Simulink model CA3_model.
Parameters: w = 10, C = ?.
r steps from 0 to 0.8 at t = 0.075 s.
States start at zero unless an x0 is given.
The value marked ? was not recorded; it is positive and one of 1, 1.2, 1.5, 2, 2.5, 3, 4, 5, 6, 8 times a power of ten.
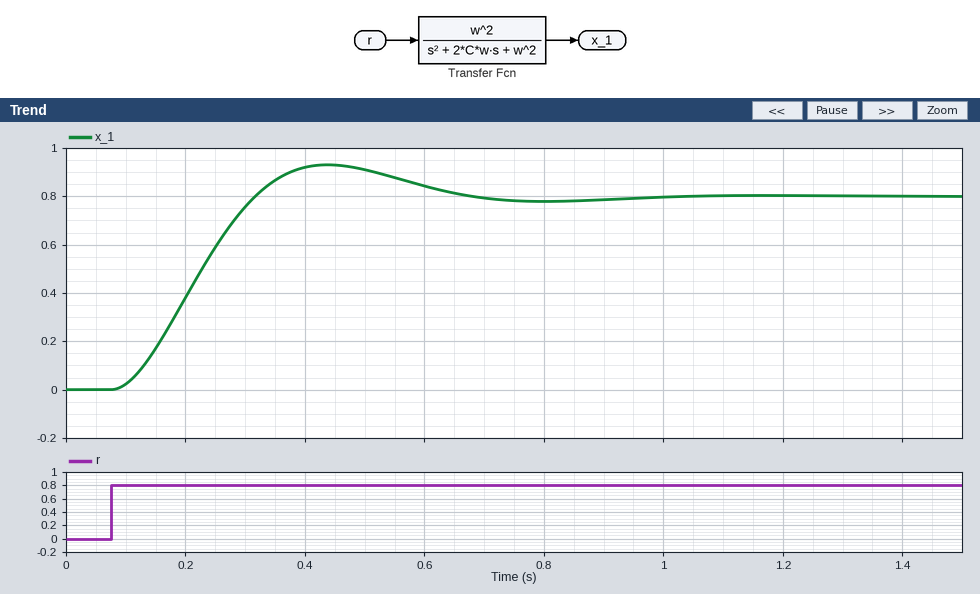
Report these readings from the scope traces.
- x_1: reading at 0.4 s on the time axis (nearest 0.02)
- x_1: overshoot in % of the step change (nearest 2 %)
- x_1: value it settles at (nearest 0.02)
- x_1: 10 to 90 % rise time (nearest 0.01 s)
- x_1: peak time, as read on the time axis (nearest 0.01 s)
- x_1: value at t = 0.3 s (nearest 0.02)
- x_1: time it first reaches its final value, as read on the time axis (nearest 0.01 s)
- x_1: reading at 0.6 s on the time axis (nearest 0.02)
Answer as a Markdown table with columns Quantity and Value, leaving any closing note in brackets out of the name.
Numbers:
| Quantity | Value |
|---|---|
| x_1: reading at 0.4 s on the time axis | 0.92 |
| x_1: overshoot in % of the step change | 16 % |
| x_1: value it settles at | 0.80 |
| x_1: 10 to 90 % rise time | 0.16 s |
| x_1: peak time, as read on the time axis | 0.44 s |
| x_1: value at t = 0.3 s | 0.76 |
| x_1: time it first reaches its final value, as read on the time axis | 0.32 s |
| x_1: reading at 0.6 s on the time axis | 0.84 |
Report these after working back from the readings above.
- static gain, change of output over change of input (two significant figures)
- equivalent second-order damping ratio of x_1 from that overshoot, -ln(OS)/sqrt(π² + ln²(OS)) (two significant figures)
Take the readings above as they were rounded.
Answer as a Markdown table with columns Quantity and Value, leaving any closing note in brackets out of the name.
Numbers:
| Quantity | Value |
|---|---|
| static gain, change of output over change of input | 1.0 |
| equivalent second-order damping ratio of x_1 from that overshoot, -ln(OS)/sqrt(π² + ln²(OS)) | 0.50 |
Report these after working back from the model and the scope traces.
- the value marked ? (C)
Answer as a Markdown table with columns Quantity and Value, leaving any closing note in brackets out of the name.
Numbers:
| Quantity | Value |
|---|---|
| the value marked ? | 0.5 |
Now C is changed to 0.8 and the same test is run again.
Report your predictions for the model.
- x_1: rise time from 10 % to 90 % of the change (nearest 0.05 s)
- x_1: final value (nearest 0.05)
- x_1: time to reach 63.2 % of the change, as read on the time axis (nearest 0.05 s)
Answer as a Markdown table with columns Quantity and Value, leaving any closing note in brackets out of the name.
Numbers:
| Quantity | Value |
|---|---|
| x_1: rise time from 10 % to 90 % of the change | 0.25 s |
| x_1: final value | 0.80 |
| x_1: time to reach 63.2 % of the change, as read on the time axis | 0.25 s |
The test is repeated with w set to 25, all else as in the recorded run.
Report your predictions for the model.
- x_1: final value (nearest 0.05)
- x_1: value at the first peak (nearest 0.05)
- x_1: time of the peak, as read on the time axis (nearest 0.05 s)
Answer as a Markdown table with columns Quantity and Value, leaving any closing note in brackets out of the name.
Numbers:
| Quantity | Value |
|---|---|
| x_1: final value | 0.80 |
| x_1: value at the first peak | 0.95 |
| x_1: time of the peak, as read on the time axis | 0.20 s |
